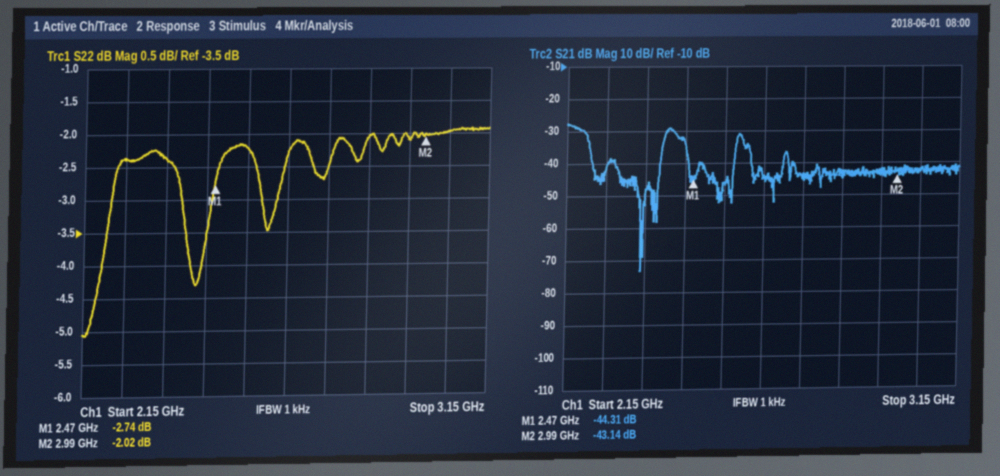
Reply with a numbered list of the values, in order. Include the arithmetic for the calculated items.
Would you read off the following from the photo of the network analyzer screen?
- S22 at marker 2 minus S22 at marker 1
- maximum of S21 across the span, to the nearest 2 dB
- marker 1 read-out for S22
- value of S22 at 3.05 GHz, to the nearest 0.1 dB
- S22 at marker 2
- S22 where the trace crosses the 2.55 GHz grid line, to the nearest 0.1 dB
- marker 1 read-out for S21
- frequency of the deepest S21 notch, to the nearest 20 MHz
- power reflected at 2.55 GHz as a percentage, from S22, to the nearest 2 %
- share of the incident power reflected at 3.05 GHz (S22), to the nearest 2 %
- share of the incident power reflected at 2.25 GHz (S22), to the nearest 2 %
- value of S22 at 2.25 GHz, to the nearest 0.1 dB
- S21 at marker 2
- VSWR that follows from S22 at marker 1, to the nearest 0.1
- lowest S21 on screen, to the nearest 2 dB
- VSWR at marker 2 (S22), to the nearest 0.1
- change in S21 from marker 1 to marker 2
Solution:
1. -2.02 − (-2.74) = 0.72 dB
2. -28 dB
3. -2.74 dB
4. -2.0 dB
5. -2.02 dB
6. -2.2 dB
7. -44.31 dB
8. 2.34 GHz
9. 10^(-2.2/10) ≈ 60 %
10. 10^(-2/10) ≈ 63.1 %, so 64 % to the nearest 2 %
11. 10^(-2.4/10) ≈ 58 %
12. -2.4 dB
13. -43.14 dB
14. (1 + 0.7295)/(1 − 0.7295) ≈ 6.4
15. -74 dB
16. (1 + 0.7925)/(1 − 0.7925) ≈ 8.6
17. -43.14 − (-44.31) = 1.17 dB
